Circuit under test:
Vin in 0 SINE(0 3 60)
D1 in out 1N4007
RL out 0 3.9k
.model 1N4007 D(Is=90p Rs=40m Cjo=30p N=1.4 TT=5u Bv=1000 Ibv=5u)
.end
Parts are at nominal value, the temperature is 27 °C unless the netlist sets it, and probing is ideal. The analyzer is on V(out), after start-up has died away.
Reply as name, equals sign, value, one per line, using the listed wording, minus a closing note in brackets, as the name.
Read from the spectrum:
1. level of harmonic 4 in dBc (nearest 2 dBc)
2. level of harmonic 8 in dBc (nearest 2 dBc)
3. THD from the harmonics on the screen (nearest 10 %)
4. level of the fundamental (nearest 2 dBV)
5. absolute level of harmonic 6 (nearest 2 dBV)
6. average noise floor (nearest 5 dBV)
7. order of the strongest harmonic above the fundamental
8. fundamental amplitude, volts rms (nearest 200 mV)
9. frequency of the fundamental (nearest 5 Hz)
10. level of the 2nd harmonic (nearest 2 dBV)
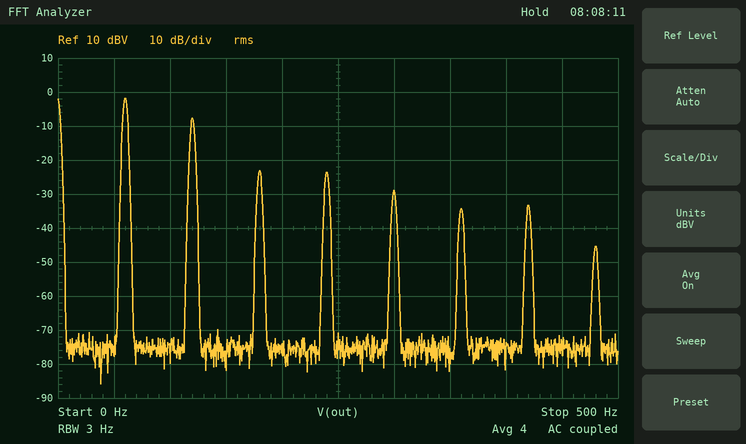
level of harmonic 4 in dBc = -22 dBc
level of harmonic 8 in dBc = -44 dBc
THD from the harmonics on the screen = 50 %
level of the fundamental = -2 dBV
absolute level of harmonic 6 = -34 dBV
average noise floor = -75 dBV
order of the strongest harmonic above the fundamental = 2
fundamental amplitude, volts rms = 800 mV
frequency of the fundamental = 60 Hz
level of the 2nd harmonic = -8 dBV
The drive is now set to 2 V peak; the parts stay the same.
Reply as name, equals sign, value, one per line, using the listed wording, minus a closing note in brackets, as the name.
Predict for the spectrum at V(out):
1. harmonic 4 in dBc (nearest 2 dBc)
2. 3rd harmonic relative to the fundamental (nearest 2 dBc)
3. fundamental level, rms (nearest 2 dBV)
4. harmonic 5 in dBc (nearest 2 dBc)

harmonic 4 in dBc = -24 dBc
3rd harmonic relative to the fundamental = -18 dBc
fundamental level, rms = -6 dBV
harmonic 5 in dBc = -24 dBc
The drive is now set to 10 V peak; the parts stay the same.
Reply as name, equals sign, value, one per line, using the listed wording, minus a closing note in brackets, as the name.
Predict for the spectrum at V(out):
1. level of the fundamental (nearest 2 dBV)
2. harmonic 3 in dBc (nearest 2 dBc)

level of the fundamental = 10 dBV
harmonic 3 in dBc = -32 dBc
